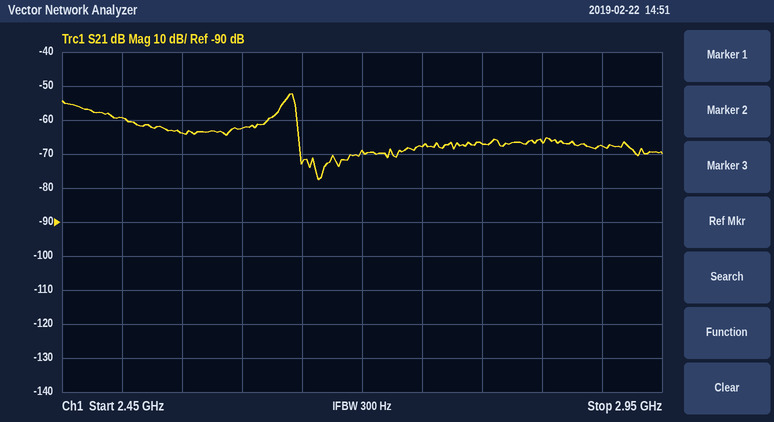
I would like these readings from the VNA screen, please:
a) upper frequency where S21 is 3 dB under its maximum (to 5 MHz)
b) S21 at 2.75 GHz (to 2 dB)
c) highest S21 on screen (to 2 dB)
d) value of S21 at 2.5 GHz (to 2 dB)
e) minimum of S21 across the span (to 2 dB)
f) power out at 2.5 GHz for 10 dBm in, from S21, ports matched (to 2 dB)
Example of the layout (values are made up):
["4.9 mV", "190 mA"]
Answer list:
["2.645 GHz", "-68 dB", "-52 dB", "-60 dB", "-78 dB", "-50 dBm"]
